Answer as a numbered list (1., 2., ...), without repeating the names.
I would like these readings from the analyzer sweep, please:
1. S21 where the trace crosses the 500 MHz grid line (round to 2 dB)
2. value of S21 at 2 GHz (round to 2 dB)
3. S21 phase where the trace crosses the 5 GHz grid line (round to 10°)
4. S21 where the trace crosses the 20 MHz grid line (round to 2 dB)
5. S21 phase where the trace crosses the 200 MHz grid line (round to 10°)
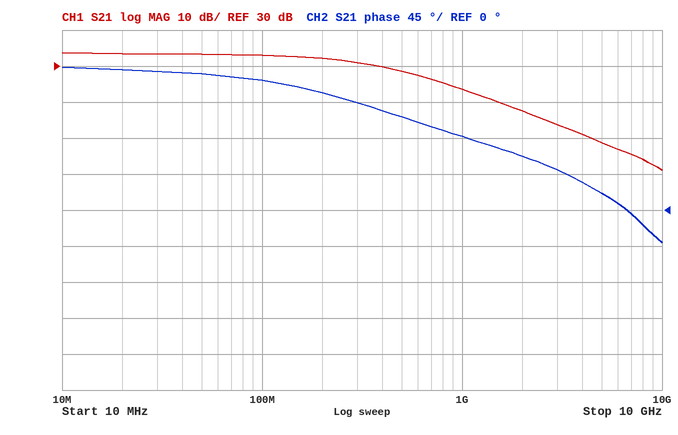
1. 28 dB
2. 18 dB
3. 20°
4. 34 dB
5. 150°
